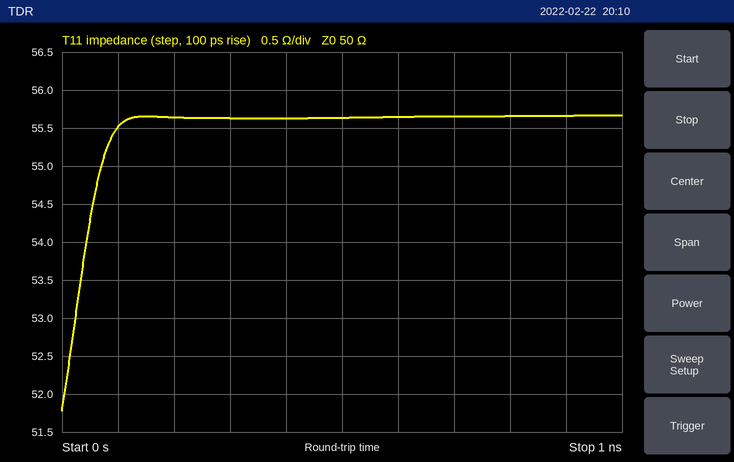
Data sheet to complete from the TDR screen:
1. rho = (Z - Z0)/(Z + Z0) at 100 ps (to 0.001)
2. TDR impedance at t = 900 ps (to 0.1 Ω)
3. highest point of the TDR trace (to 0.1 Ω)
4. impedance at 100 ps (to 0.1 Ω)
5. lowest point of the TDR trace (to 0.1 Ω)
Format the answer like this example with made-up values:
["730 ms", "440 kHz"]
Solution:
["+0.052", "55.7 Ω", "55.7 Ω", "55.5 Ω", "51.8 Ω"]
